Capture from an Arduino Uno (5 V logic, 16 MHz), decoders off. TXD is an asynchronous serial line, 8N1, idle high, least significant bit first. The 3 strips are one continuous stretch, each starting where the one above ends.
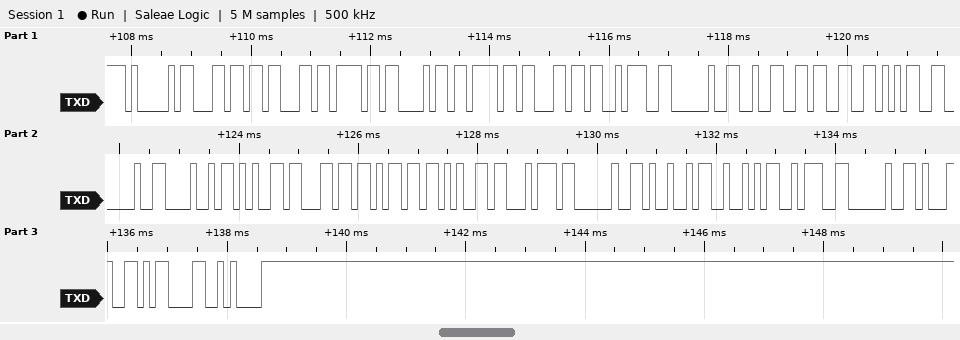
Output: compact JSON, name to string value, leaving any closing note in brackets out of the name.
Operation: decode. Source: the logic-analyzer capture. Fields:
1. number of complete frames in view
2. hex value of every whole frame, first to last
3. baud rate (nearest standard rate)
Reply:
{"number of complete frames in view": "27", "hex value of every whole frame, first to last": "0x41 0x6C 0x63 0x6F 0x68 0x6F 0x6C 0x3A 0x20 0x32 0x33 0x35 0x20 0x48 0x65 0x6C 0x6D 0x65 0x74 0x20 0x49 0x52 0x3A 0x20 0x31 0x0D 0x0A", "baud rate": "9600 baud"}
